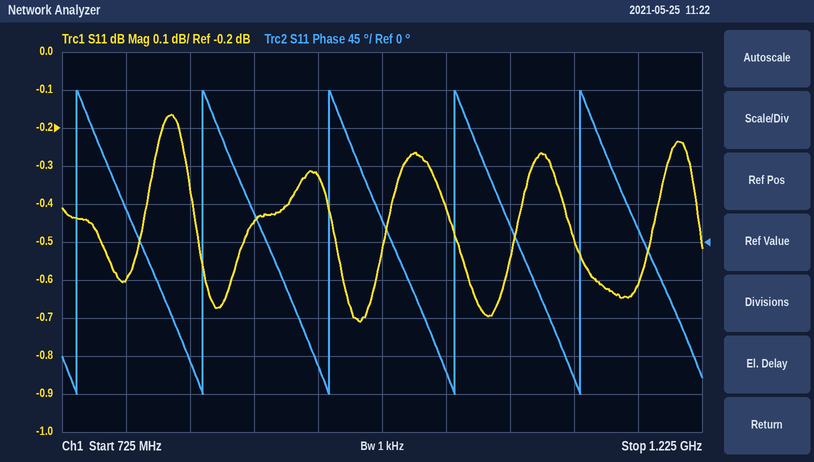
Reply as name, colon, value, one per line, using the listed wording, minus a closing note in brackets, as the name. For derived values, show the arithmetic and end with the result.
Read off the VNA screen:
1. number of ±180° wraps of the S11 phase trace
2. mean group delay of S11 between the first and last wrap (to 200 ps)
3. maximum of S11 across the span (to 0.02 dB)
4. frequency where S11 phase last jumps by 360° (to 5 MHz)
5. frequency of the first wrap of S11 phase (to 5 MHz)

number of ±180° wraps of the S11 phase trace: 5
mean group delay of S11 between the first and last wrap: 4 cycles / (1.130 GHz − 735 MHz) ≈ 10.1 ns, so 10.2 ns to the nearest 200 ps
maximum of S11 across the span: -0.16 dB
frequency where S11 phase last jumps by 360°: 1.130 GHz
frequency of the first wrap of S11 phase: 735 MHz
